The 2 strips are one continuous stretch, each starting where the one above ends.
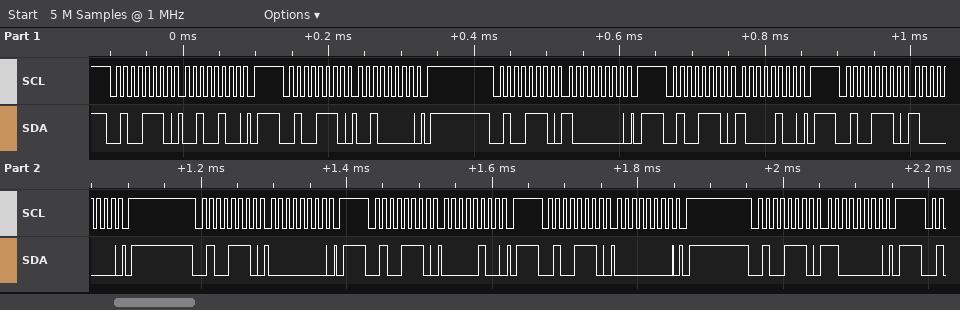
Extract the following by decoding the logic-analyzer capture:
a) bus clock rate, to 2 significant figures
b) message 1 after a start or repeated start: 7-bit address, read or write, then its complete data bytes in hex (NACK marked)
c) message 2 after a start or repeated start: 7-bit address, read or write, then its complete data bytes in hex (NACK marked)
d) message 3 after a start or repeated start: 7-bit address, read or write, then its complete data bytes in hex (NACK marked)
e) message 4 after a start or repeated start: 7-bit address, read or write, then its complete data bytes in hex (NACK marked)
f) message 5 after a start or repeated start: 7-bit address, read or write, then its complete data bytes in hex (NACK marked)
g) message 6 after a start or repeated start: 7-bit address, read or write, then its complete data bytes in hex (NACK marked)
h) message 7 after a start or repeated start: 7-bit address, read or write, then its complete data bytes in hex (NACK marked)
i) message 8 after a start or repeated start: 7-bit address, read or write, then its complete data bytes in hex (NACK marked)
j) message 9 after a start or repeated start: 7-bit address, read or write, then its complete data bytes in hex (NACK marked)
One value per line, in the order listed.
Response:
100 kHz
0x27 write: 24
0x27 write: 20
0x27 write: 80
0x27 write: 84
0x27 write: 80
0x27 write: 00
0x27 write: 04
0x27 write: 00
0x27 write: C0
